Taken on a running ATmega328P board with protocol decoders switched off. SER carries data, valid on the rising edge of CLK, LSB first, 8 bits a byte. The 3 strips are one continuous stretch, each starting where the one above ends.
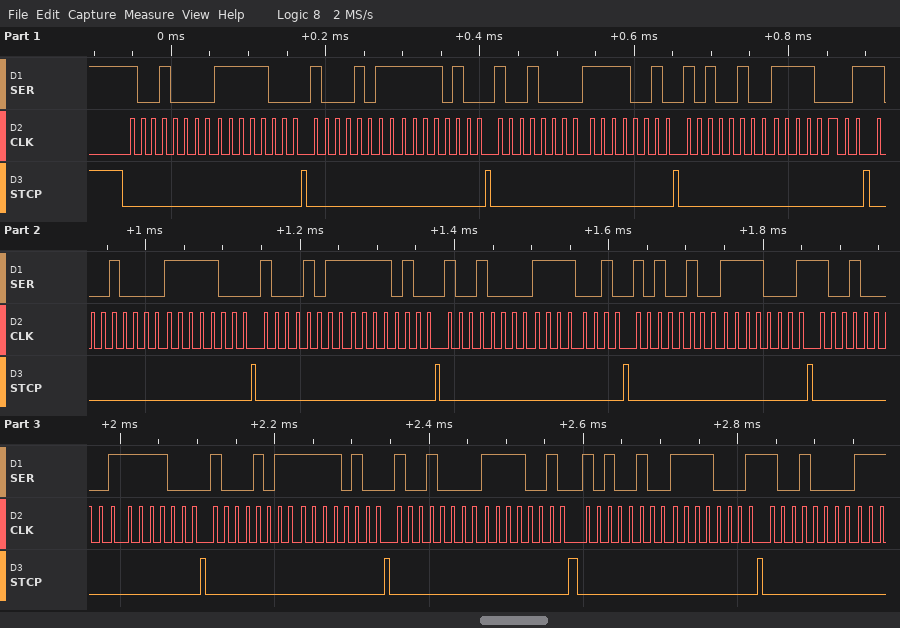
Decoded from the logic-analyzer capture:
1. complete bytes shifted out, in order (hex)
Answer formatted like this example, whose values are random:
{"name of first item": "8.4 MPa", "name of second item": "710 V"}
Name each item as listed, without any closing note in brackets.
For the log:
{"complete bytes shifted out, in order": "0x09 0x1F 0xD1 0x2F 0x09 0x4F 0x25 0x8F 0x09 0x1F 0xD1 0x2F 0x09 0x4F 0x25 0x8F 0x09 0x1F 0xD1 0x2F 0x09 0x4F 0x25 0x8F 0x09"}
